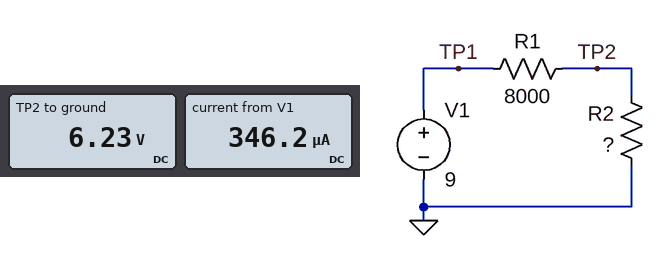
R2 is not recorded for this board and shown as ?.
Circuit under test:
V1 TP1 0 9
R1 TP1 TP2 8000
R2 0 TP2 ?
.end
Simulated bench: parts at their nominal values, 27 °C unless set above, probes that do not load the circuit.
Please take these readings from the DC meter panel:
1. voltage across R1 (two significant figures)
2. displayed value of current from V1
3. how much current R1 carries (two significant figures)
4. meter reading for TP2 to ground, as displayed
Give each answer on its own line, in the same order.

2.8 V
346.2 µA
350 µA
6.23 V
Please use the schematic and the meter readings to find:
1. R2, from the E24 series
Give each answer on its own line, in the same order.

18 kΩ
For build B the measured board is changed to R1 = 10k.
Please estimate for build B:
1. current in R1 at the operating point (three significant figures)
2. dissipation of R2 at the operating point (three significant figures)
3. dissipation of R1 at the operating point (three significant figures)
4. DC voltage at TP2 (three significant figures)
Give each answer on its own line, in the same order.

321 µA
1.86 mW
1.03 mW
5.79 V
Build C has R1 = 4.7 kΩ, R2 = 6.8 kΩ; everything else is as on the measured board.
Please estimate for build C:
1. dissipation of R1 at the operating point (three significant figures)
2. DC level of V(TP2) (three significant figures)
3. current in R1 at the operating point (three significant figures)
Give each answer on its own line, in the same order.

2.88 mW
5.32 V
783 µA
